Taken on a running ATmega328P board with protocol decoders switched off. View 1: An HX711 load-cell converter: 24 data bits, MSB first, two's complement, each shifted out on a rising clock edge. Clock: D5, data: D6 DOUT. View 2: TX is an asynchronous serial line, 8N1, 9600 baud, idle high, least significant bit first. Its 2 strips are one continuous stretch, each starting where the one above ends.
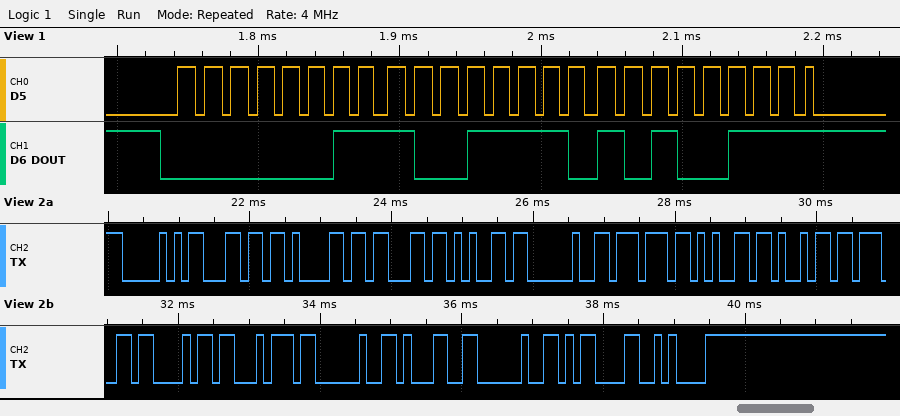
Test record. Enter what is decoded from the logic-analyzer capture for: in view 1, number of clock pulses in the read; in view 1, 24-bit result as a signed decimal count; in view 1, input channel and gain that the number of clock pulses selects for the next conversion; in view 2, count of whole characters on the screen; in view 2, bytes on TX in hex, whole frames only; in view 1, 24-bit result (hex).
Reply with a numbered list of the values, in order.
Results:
1. 25
2. 237223
3. channel A, gain 128
4. 17
5. 50 6C 61 63 65 20 77 65 69 67 68 74 20 31 20 0D 0A
6. 0x039EA7
